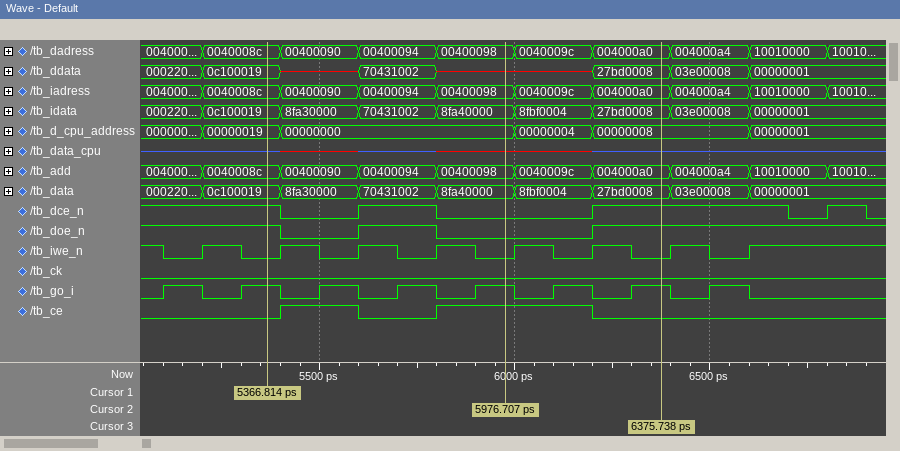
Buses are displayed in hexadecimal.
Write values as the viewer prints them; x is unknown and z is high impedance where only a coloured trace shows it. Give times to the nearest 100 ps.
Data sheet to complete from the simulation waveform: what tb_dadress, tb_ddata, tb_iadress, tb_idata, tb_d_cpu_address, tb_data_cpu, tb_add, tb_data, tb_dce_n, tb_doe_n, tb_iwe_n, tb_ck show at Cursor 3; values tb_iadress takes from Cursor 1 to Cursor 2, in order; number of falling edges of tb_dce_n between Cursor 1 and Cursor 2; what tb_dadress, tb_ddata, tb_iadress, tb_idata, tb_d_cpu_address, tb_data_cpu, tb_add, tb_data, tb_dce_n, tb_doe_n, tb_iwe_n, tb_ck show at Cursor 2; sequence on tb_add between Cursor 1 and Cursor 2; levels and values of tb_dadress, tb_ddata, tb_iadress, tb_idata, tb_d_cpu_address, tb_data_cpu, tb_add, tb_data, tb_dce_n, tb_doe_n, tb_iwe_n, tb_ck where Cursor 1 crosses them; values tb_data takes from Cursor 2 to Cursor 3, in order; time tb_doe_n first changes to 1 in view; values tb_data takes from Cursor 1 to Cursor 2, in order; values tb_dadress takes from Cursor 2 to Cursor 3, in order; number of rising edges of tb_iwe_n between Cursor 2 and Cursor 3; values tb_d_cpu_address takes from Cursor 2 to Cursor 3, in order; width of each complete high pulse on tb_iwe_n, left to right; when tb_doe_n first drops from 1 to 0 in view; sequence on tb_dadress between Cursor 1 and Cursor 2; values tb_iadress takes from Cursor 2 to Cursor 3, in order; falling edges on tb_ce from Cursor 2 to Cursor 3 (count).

tb_dadress=004000a0, tb_ddata=27bd0008, tb_iadress=004000a0, tb_idata=27bd0008, tb_d_cpu_address=00000008, tb_data_cpu=z, tb_add=004000a0, tb_data=27bd0008, tb_dce_n=1, tb_doe_n=1, tb_iwe_n=0, tb_ck=0
0040008c, 00400090, 00400094, 00400098
2
tb_dadress=00400098, tb_ddata=x, tb_iadress=00400098, tb_idata=8fa40000, tb_d_cpu_address=00000000, tb_data_cpu=x, tb_add=00400098, tb_data=8fa40000, tb_dce_n=0, tb_doe_n=0, tb_iwe_n=0, tb_ck=0
0040008c, 00400090, 00400094, 00400098
tb_dadress=0040008c, tb_ddata=0c100019, tb_iadress=0040008c, tb_idata=0c100019, tb_d_cpu_address=00000019, tb_data_cpu=z, tb_add=0040008c, tb_data=0c100019, tb_dce_n=1, tb_doe_n=1, tb_iwe_n=0, tb_ck=0
8fa40000, 8fbf0004, 27bd0008
5600 ps
0c100019, 8fa30000, 70431002, 8fa40000
00400098, 0040009c, 004000a0
2
00000000, 00000004, 00000008
100 ps, 100 ps, 100 ps, 100 ps, 100 ps, 100 ps, 100 ps
5400 ps
0040008c, 00400090, 00400094, 00400098
00400098, 0040009c, 004000a0
1
